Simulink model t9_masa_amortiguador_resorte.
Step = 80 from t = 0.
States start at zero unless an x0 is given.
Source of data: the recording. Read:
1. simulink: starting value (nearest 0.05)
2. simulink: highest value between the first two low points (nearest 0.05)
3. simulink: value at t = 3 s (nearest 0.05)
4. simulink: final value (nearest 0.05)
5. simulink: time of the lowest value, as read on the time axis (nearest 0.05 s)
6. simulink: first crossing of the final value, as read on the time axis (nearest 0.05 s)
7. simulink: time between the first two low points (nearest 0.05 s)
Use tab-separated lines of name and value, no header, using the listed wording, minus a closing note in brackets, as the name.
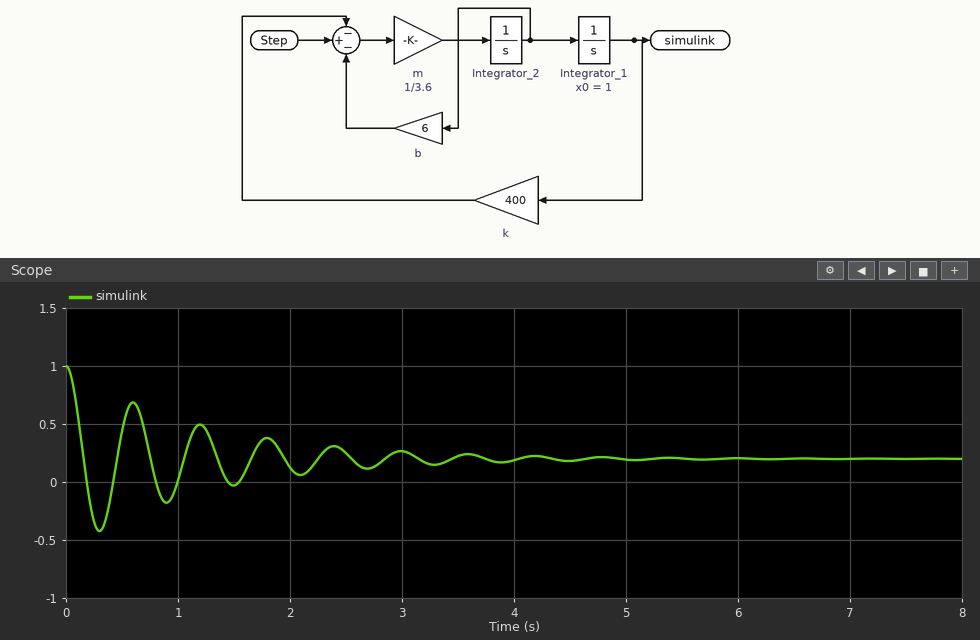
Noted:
simulink: starting value	1.00
simulink: highest value between the first two low points	0.70
simulink: value at t = 3 s	0.25
simulink: final value	0.20
simulink: time of the lowest value, as read on the time axis	0.30 s
simulink: first crossing of the final value, as read on the time axis	0.15 s
simulink: time between the first two low points	0.60 s
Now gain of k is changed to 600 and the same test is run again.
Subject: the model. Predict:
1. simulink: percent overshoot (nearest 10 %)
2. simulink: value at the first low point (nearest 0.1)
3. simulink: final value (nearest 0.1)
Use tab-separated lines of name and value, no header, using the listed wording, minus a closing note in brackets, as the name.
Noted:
simulink: percent overshoot	80 %
simulink: value at the first low point	-0.6
simulink: final value	0.1
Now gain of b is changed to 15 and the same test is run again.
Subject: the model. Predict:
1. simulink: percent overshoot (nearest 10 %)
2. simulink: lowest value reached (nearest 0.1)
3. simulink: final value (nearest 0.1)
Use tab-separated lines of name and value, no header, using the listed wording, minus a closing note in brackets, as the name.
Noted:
simulink: percent overshoot	50 %
simulink: lowest value reached	-0.2
simulink: final value	0.2
